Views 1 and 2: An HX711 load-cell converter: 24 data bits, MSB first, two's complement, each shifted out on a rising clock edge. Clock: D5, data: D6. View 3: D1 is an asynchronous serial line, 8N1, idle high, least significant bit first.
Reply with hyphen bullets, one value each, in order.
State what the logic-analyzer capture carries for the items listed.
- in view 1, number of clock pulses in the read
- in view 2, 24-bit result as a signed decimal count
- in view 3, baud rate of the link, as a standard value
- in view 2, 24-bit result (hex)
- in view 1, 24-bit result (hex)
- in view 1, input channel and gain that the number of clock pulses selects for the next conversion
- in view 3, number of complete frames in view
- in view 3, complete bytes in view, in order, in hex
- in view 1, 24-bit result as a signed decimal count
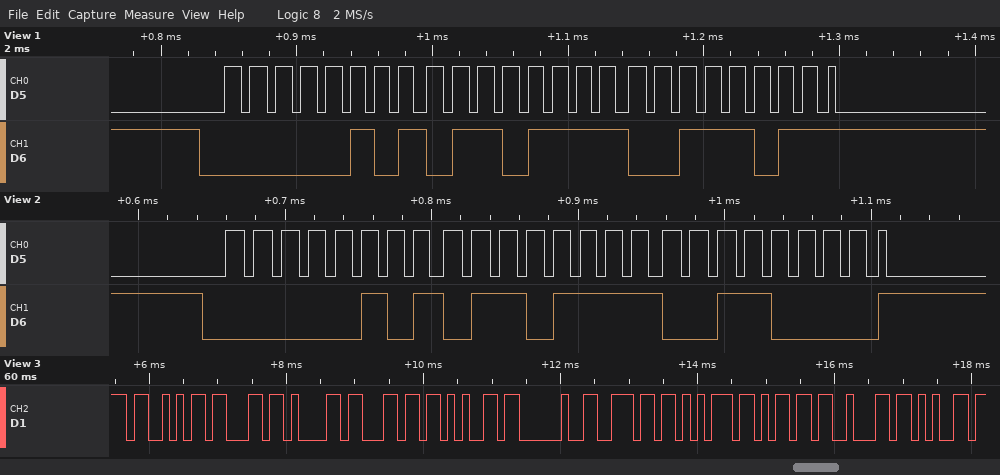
- 25
- 356144
- 9600 baud
- 0x056F30
- 0x056F3B
- channel A, gain 128
- 11
- 53 63 61 6C 65 20 6E 75 6D 62 65
- 356155
